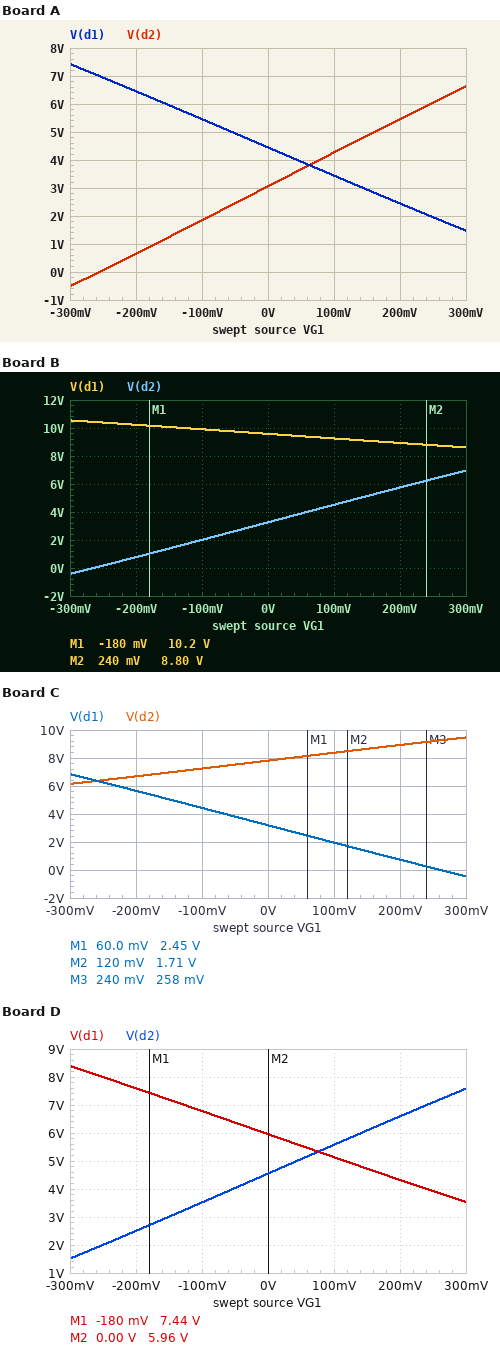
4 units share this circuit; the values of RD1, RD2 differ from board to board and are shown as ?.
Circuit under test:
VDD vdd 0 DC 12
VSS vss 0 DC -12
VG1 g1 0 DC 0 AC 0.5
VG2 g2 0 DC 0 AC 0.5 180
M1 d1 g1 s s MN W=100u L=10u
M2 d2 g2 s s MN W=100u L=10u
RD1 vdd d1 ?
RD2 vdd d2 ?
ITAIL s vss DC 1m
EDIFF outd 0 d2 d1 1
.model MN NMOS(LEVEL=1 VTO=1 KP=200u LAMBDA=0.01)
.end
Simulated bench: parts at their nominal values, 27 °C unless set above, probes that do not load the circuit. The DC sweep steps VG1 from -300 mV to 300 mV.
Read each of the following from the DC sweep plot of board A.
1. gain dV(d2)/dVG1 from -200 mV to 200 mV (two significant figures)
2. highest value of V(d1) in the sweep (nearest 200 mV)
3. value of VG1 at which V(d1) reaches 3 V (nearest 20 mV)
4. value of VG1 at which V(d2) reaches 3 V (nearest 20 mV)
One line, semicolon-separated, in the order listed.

12 V/V; 7.4 V; 140 mV; 0 V
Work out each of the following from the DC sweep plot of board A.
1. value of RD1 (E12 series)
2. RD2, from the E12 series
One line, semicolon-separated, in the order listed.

15 kΩ; 18 kΩ
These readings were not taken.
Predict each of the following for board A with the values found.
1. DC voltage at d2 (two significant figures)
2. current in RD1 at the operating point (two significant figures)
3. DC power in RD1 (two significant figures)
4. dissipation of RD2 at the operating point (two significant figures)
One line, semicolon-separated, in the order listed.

3.1 V; 500 µA; 3.8 mW; 4.4 mW
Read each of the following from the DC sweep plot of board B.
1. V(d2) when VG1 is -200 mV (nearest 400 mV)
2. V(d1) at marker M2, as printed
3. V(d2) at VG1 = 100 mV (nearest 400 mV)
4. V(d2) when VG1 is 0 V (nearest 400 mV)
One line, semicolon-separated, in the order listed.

800 mV; 8.80 V; 4.4 V; 3.2 V
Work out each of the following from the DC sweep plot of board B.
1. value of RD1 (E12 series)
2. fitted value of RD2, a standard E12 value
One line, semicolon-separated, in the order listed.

4.7 kΩ; 18 kΩ
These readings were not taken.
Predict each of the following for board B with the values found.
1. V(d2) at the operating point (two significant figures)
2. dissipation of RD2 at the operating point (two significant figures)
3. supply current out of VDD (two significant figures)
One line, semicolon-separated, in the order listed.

3.3 V; 4.2 mW; 1.0 mA
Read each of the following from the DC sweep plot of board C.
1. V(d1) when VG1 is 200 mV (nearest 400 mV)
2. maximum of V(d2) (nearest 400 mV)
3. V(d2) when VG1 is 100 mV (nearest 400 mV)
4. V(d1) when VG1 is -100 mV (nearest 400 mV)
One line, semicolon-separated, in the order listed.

800 mV; 9.6 V; 8.4 V; 4.4 V
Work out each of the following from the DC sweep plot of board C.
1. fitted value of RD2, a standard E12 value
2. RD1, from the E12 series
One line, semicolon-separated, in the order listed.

8.2 kΩ; 18 kΩ
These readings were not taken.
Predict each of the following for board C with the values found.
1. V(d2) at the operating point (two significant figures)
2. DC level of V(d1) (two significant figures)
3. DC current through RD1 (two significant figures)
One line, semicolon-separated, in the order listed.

7.8 V; 3.2 V; 490 µA
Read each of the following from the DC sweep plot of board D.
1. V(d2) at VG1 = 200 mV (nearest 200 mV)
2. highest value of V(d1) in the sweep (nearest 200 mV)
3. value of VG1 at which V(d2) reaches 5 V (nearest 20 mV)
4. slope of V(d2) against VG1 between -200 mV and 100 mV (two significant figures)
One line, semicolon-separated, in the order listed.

6.6 V; 8.4 V; 40 mV; 10 V/V
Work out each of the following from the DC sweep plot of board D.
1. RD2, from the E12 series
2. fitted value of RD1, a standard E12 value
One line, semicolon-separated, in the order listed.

15 kΩ; 12 kΩ
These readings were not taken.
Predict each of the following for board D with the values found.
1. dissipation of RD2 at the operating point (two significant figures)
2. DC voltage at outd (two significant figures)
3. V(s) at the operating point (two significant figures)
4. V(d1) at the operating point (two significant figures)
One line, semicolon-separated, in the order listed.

3.7 mW; -1.4 V; -1.7 V; 6.0 V
